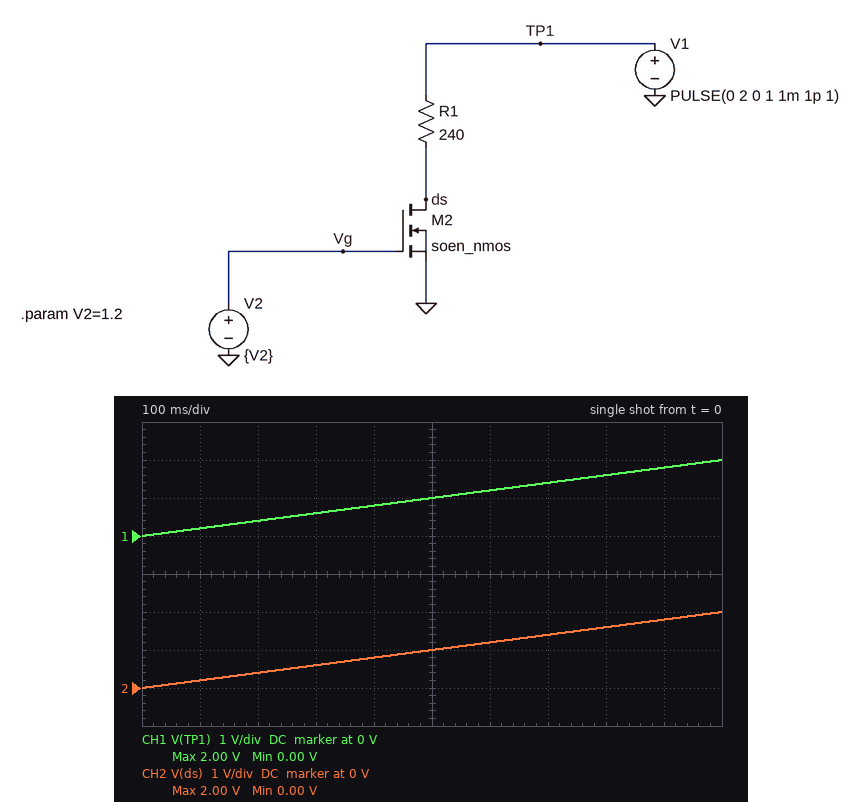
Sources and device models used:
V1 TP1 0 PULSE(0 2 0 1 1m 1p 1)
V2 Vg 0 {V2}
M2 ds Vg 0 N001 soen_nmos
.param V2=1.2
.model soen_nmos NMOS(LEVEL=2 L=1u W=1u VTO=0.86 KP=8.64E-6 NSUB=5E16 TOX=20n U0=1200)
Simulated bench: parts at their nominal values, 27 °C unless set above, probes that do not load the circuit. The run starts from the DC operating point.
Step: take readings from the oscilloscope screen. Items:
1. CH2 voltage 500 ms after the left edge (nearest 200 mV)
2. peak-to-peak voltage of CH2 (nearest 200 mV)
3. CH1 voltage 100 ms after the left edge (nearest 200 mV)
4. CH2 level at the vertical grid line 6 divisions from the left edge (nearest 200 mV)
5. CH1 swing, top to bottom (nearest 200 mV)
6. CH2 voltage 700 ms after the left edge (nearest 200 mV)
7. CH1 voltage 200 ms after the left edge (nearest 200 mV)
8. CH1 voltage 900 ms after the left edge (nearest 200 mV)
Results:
1.0 V
2.0 V
200 mV
1.2 V
2.0 V
1.4 V
400 mV
1.8 V
